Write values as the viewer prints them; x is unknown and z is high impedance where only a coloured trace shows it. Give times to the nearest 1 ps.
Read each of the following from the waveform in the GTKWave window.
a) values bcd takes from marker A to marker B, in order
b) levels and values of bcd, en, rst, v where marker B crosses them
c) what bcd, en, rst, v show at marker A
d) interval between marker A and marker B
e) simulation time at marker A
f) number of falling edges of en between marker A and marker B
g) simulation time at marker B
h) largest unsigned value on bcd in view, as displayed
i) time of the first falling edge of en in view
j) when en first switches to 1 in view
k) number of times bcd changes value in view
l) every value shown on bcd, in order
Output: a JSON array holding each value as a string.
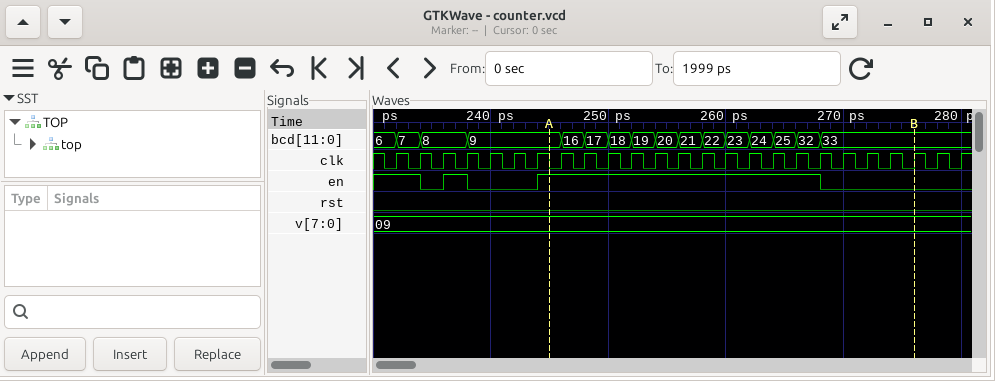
["9, 16, 17, 18, 19, 20, 21, 22, 23, 24, 25, 32, 33", "bcd=33, en=0, rst=0, v=09", "bcd=9, en=1, rst=0, v=09", "31 ps", "245 ps", "1", "276 ps", "33", "234 ps", "236 ps", "15", "6, 7, 8, 9, 16, 17, 18, 19, 20, 21, 22, 23, 24, 25, 32, 33"]
